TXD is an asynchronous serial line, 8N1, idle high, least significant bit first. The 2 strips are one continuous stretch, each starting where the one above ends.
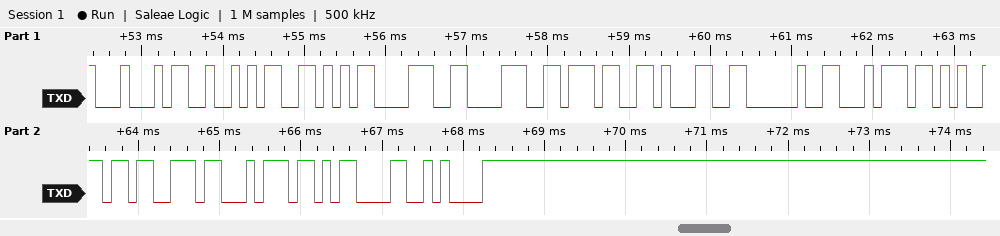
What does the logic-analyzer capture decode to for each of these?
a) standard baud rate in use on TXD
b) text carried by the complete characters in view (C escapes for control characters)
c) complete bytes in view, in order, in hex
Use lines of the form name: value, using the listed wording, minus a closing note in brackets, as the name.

standard baud rate in use on TXD: 9600 baud
text carried by the complete characters in view: "DRV8871 test\r\n"
complete bytes in view, in order, in hex: 0x44 0x52 0x56 0x38 0x38 0x37 0x31 0x20 0x74 0x65 0x73 0x74 0x0D 0x0A
